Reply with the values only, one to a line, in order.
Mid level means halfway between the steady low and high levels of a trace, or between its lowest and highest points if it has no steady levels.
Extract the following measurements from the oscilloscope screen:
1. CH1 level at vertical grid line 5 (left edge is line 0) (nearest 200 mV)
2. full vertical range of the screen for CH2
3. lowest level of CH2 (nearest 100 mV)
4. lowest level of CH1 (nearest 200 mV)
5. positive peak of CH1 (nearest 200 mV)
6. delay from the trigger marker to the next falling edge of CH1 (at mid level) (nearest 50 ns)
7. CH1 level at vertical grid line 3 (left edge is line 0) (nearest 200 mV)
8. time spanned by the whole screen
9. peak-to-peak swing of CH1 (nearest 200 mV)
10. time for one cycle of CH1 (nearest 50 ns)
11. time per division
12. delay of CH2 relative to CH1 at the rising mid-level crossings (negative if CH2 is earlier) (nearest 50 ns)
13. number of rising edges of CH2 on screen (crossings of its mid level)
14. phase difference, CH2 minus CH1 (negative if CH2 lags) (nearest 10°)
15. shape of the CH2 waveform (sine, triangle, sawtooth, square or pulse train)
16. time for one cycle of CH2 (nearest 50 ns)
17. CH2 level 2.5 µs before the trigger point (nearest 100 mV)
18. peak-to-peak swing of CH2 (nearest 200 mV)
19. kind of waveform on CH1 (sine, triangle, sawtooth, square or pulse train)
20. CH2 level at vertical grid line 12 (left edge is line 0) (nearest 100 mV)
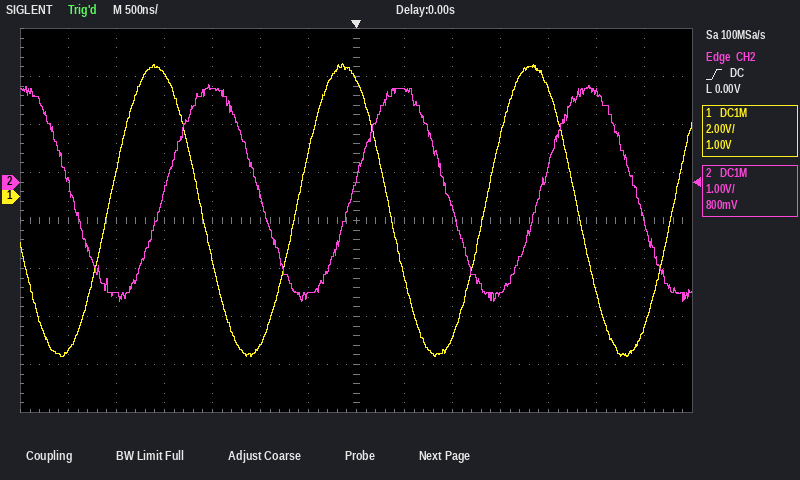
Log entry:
-6.2 V
8 V
-2.5 V
-6.6 V
5.6 V
350 ns
5.2 V
7 µs
12.2 V
1.95 µs
500 ns
+600 ns
3
-110°
sine
1.95 µs
-2.3 V
4.6 V
sine
1.9 V
